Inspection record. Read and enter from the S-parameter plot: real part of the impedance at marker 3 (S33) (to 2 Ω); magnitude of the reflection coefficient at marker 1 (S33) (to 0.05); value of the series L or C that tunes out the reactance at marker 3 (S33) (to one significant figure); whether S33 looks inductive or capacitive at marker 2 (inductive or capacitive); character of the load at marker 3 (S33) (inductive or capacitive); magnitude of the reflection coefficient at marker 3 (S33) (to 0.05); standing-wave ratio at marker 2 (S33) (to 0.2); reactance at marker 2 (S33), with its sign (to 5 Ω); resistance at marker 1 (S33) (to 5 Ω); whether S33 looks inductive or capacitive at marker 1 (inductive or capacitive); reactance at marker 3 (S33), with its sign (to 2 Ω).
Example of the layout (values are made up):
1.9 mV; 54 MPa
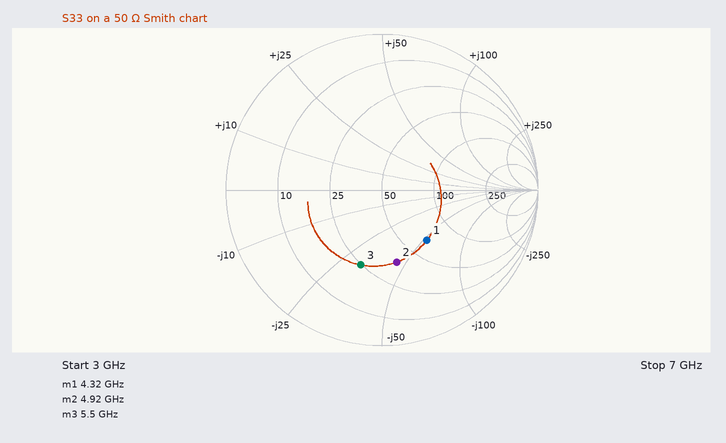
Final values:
24 Ω; 0.45; 900 pH; capacitive; capacitive; 0.50; 2.8; -45 Ω; 65 Ω; capacitive; -32 Ω
